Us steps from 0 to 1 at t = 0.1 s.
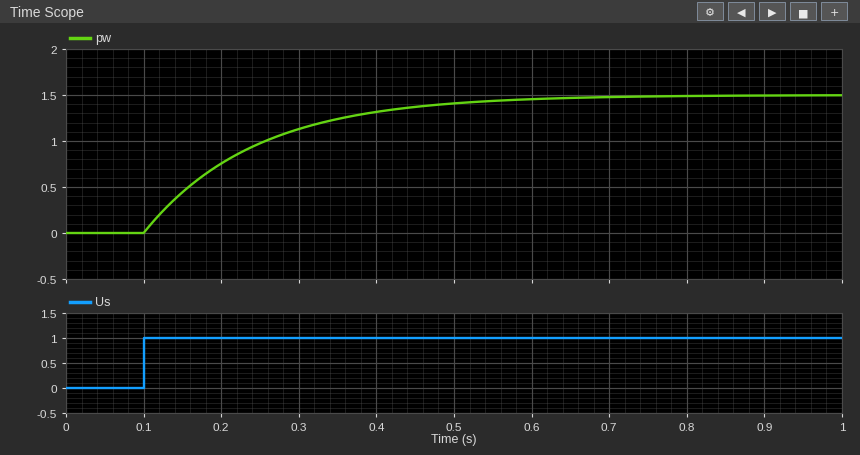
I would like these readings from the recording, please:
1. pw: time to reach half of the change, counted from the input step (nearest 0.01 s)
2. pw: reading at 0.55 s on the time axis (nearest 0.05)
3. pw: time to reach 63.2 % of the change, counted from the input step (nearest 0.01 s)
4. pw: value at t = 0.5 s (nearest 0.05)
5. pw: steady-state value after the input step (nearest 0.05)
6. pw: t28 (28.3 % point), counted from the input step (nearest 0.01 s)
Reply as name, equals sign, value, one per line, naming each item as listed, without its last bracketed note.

pw: time to reach half of the change, counted from the input step = 0.10 s
pw: reading at 0.55 s on the time axis = 1.45
pw: time to reach 63.2 % of the change, counted from the input step = 0.14 s
pw: value at t = 0.5 s = 1.40
pw: steady-state value after the input step = 1.50
pw: t28 (28.3 % point), counted from the input step = 0.05 s
